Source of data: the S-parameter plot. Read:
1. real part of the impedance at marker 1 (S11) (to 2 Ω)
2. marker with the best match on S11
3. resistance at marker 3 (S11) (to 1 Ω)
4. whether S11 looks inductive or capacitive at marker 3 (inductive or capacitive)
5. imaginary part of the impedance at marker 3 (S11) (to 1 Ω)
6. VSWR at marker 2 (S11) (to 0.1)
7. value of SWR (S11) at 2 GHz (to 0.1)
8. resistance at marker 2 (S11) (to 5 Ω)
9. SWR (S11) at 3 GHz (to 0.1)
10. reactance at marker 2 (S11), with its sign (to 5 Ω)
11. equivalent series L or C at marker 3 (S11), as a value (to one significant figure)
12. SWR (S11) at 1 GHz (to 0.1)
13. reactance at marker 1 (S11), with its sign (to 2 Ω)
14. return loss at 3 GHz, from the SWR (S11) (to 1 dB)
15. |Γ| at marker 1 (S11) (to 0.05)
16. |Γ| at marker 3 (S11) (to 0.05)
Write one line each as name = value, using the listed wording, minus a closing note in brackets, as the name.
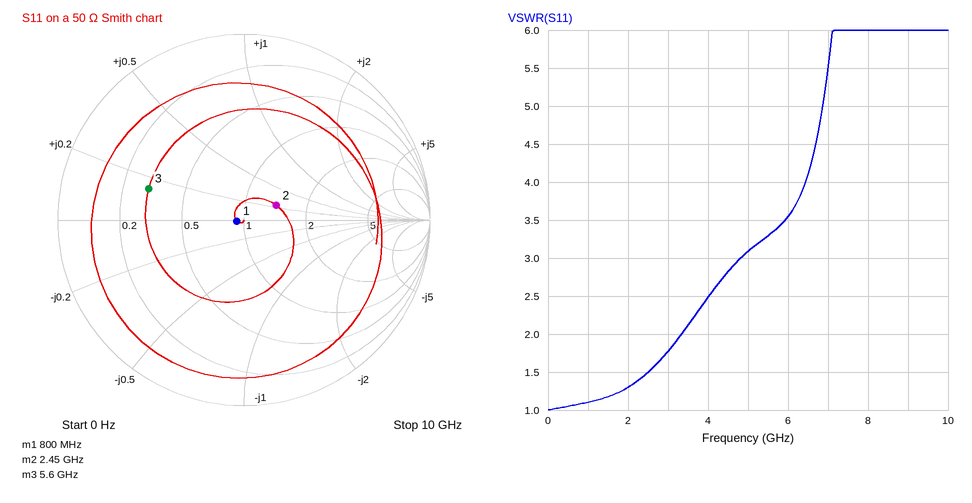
real part of the impedance at marker 1 (S11) = 46 Ω
marker with the best match on S11 = marker 1
resistance at marker 3 (S11) = 15 Ω
whether S11 looks inductive or capacitive at marker 3 = inductive
imaginary part of the impedance at marker 3 (S11) = +7 Ω
VSWR at marker 2 (S11) = 1.5
value of SWR (S11) at 2 GHz = 1.3
resistance at marker 2 (S11) = 70 Ω
SWR (S11) at 3 GHz = 1.8
reactance at marker 2 (S11), with its sign = +10 Ω
equivalent series L or C at marker 3 (S11), as a value = 200 pH
SWR (S11) at 1 GHz = 1.1
reactance at marker 1 (S11), with its sign = 0 Ω
return loss at 3 GHz, from the SWR (S11) = 11 dB
|Γ| at marker 1 (S11) = 0.05
|Γ| at marker 3 (S11) = 0.55
